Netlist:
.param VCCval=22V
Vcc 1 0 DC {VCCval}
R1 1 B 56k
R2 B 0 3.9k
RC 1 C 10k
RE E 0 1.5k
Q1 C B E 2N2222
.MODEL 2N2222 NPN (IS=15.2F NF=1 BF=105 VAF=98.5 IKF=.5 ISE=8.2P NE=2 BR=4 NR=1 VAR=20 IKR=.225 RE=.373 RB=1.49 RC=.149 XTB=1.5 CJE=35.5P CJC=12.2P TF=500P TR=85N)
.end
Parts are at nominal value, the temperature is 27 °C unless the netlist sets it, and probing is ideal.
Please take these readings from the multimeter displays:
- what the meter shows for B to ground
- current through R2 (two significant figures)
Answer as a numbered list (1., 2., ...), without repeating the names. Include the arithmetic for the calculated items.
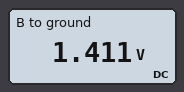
1. 1.411 V
2. (1.411 V) / 3.9 kΩ = 360 µA
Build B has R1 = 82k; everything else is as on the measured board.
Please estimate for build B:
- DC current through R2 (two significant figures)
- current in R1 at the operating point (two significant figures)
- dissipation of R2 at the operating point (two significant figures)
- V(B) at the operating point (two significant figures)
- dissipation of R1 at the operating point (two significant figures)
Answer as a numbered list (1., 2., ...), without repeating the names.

1. 250 µA
2. 260 µA
3. 250 µW
4. 990 mV
5. 5.4 mW
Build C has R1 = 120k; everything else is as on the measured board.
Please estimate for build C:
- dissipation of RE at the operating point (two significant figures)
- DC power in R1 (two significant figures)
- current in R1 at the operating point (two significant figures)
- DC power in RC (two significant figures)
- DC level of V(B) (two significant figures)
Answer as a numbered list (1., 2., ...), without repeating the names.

1. 8.8 µW
2. 3.8 mW
3. 180 µA
4. 57 µW
5. 690 mV
